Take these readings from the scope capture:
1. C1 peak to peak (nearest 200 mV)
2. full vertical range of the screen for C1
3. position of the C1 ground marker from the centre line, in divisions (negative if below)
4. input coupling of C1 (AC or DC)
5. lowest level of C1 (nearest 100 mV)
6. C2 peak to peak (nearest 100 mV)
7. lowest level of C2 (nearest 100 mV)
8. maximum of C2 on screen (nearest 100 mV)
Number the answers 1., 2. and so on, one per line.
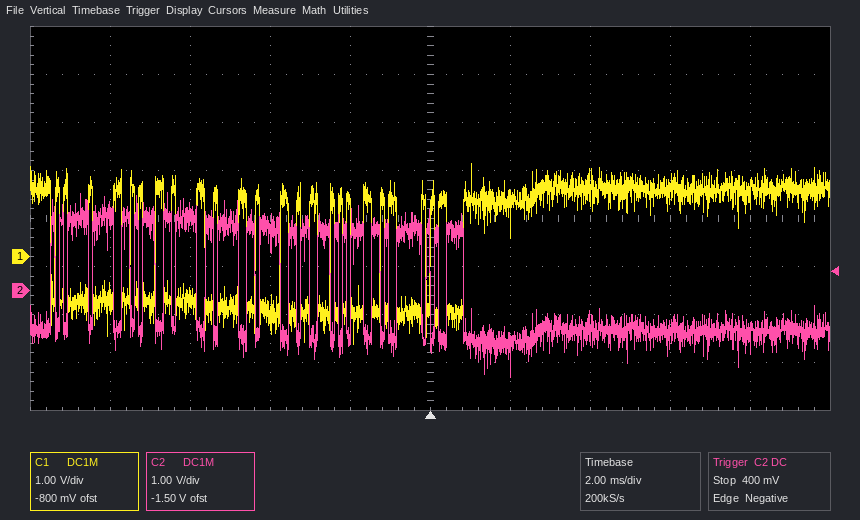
1. 3.8 V
2. 8 V
3. -0.8 div
4. DC
5. -1.8 V
6. 3.8 V
7. -1.8 V
8. 2.0 V
